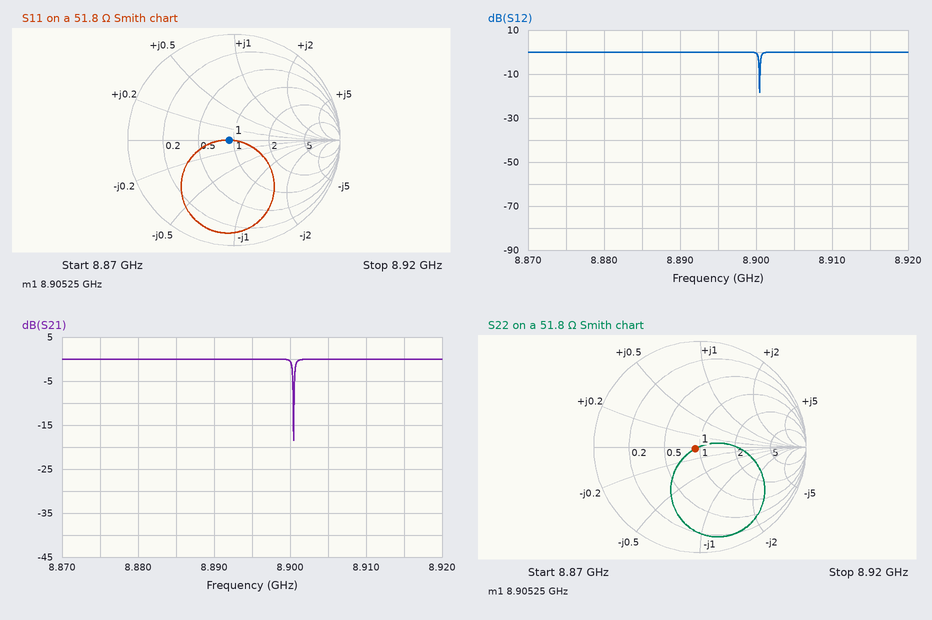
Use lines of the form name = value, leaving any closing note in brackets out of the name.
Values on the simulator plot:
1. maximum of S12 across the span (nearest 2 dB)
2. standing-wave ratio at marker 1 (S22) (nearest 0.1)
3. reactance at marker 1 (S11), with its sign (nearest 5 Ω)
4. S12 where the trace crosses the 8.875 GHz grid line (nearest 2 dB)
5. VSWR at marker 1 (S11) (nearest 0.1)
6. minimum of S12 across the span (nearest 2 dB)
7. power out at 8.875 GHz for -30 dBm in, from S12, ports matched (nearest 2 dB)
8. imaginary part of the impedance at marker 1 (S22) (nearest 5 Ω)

maximum of S12 across the span = 0 dB
standing-wave ratio at marker 1 (S22) = 1.1
reactance at marker 1 (S11), with its sign = 0 Ω
S12 where the trace crosses the 8.875 GHz grid line = 0 dB
VSWR at marker 1 (S11) = 1.1
minimum of S12 across the span = -18 dB
power out at 8.875 GHz for -30 dBm in, from S12, ports matched = -30 dBm
imaginary part of the impedance at marker 1 (S22) = 0 Ω
